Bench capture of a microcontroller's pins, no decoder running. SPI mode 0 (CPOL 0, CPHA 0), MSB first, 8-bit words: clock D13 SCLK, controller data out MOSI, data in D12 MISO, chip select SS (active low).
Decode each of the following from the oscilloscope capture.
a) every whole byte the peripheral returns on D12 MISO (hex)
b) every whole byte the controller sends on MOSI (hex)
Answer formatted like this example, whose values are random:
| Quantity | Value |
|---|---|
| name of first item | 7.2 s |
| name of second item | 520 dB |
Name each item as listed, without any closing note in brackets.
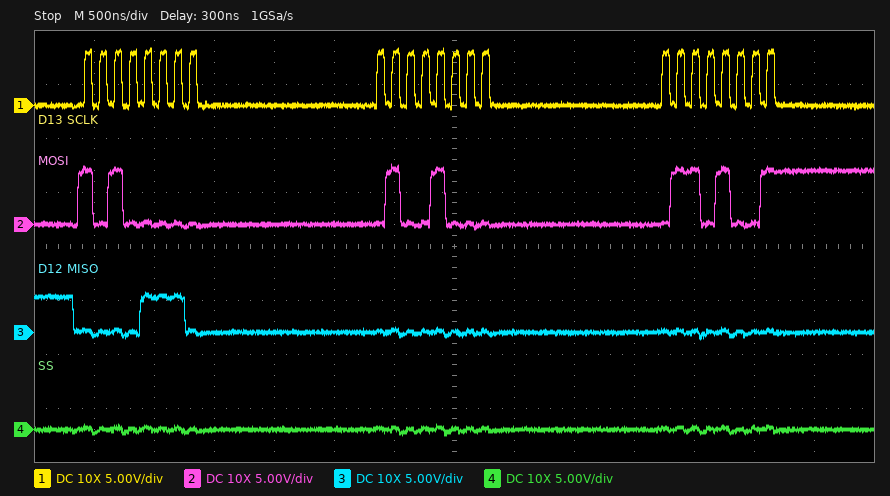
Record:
| Quantity | Value |
|---|---|
| every whole byte the peripheral returns on D12 MISO | 0E 00 00 |
| every whole byte the controller sends on MOSI | A0 48 69 |
